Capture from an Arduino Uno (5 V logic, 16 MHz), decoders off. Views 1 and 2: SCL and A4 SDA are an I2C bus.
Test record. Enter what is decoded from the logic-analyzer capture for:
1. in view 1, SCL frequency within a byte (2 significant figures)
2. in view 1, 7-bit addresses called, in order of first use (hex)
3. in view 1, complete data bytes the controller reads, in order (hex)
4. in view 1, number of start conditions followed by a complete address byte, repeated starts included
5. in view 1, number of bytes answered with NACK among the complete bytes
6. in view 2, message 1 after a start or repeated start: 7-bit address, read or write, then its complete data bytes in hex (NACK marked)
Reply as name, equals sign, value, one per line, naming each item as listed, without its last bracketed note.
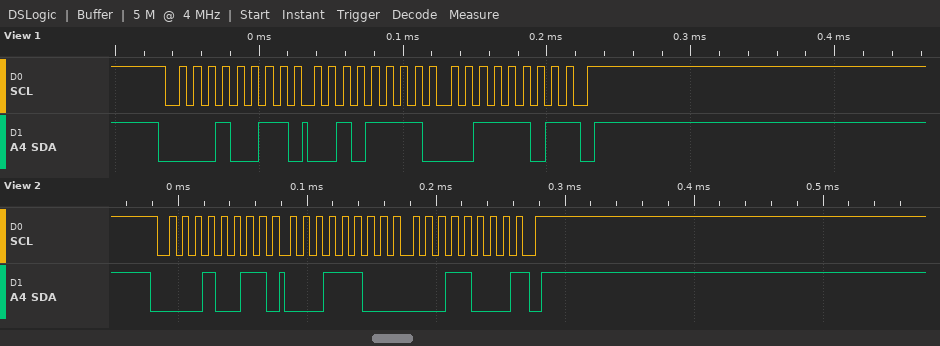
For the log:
in view 1, SCL frequency within a byte = 100 kHz
in view 1, 7-bit addresses called, in order of first use = 0x09
in view 1, complete data bytes the controller reads, in order = 2F 3D
in view 1, number of start conditions followed by a complete address byte, repeated starts included = 1
in view 1, number of bytes answered with NACK among the complete bytes = 1
in view 2, message 1 after a start or repeated start: 7-bit address, read or write, then its complete data bytes in hex = 0x09 read: 1C 18 NACK
